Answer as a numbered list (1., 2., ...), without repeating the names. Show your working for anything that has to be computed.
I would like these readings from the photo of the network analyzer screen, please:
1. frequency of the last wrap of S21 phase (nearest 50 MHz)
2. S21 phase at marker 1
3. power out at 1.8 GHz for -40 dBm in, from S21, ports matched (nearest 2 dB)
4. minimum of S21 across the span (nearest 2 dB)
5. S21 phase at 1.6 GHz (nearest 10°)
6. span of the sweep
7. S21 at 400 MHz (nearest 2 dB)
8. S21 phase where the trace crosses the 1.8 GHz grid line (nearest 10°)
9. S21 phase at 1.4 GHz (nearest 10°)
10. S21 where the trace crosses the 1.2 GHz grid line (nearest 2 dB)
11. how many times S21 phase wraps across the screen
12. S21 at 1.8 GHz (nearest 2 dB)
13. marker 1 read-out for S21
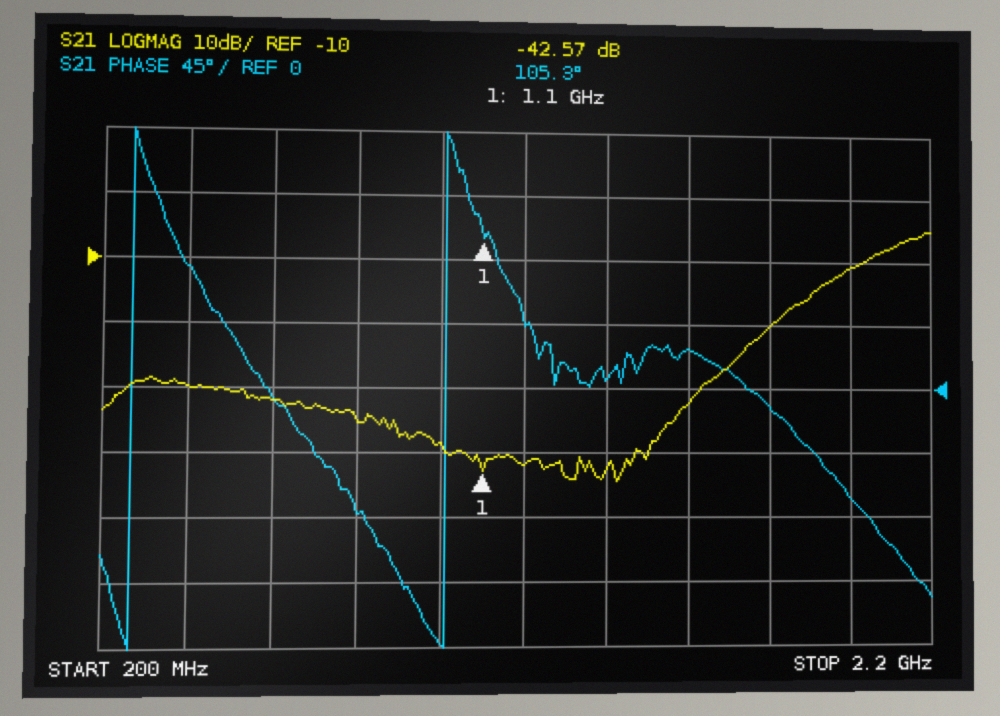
1. 1.00 GHz
2. 105.3°
3. -40 dBm + (-20 dB) = -60 dBm
4. -44 dB
5. 30°
6. 2 GHz
7. -30 dB
8. -10°
9. 10°
10. -42 dB
11. 2
12. -20 dB
13. -42.57 dB
